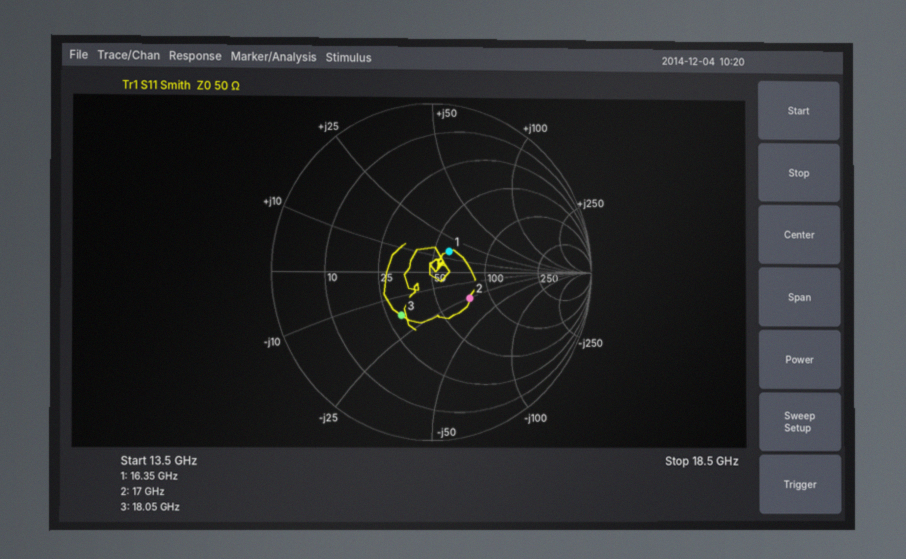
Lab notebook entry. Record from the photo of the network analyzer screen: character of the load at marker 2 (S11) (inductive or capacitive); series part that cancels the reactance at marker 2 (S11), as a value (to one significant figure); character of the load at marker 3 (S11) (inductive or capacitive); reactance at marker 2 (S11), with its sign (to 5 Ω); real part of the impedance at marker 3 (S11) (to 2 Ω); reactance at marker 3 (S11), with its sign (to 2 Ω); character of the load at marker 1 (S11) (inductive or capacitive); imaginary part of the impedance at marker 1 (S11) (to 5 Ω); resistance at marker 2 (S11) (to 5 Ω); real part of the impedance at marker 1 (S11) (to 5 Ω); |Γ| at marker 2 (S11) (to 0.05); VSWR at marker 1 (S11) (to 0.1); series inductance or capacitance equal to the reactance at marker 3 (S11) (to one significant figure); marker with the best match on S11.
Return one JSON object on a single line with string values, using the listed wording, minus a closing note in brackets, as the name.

{"character of the load at marker 2 (S11)": "capacitive", "series part that cancels the reactance at marker 2 (S11), as a value": "200 pH", "character of the load at marker 3 (S11)": "capacitive", "reactance at marker 2 (S11), with its sign": "-25 Ω", "real part of the impedance at marker 3 (S11)": "30 Ω", "reactance at marker 3 (S11), with its sign": "-18 Ω", "character of the load at marker 1 (S11)": "inductive", "imaginary part of the impedance at marker 1 (S11)": "+15 Ω", "resistance at marker 2 (S11)": "75 Ω", "real part of the impedance at marker 1 (S11)": "60 Ω", "|Γ| at marker 2 (S11)": "0.30", "VSWR at marker 1 (S11)": "1.4", "series inductance or capacitance equal to the reactance at marker 3 (S11)": "500 fF", "marker with the best match on S11": "marker 1"}
